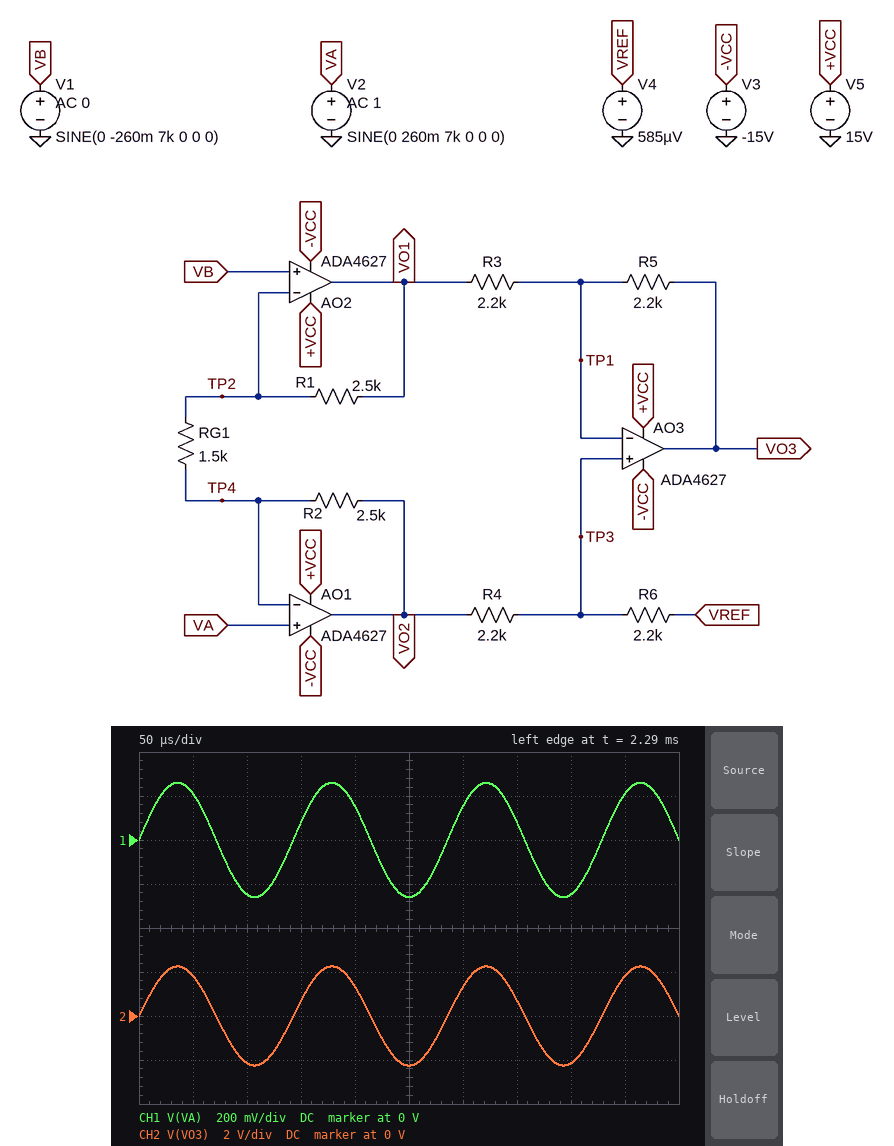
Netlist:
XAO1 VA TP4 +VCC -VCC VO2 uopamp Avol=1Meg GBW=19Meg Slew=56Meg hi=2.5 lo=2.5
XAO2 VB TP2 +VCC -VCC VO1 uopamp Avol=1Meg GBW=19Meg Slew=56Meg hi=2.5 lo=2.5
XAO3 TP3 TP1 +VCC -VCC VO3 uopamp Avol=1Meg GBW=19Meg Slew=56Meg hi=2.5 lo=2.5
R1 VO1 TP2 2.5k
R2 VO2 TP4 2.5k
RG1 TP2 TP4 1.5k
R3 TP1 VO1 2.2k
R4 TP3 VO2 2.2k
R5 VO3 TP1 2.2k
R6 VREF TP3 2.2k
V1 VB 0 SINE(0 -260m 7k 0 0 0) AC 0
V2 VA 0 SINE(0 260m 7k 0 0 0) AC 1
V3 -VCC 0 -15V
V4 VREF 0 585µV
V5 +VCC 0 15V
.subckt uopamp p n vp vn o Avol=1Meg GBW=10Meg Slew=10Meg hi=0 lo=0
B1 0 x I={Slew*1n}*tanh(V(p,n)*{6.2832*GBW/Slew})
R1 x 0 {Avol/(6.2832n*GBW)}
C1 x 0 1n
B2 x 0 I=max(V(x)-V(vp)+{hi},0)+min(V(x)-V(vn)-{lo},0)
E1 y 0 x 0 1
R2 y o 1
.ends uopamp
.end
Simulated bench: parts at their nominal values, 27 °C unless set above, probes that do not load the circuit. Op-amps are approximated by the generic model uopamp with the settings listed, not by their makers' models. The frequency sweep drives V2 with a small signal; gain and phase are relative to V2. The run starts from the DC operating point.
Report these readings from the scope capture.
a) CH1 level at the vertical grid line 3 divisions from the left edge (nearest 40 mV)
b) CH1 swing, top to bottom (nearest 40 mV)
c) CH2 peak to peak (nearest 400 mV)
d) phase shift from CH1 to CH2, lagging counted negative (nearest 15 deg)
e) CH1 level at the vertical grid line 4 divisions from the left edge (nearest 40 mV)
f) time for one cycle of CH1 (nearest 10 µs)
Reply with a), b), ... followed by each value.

a) 80 mV
b) 520 mV
c) 4.4 V
d) 0 deg
e) 160 mV
f) 140 µs
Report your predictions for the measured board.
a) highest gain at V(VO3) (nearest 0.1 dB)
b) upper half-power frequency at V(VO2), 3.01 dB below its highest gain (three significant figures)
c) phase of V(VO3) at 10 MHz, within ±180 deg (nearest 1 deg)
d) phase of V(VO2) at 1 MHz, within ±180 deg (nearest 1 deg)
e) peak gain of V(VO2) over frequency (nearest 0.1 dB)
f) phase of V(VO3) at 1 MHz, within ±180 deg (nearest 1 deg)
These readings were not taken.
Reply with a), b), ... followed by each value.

a) 12.7 dB
b) 4.79 MHz
c) -113 deg
d) -11 deg
e) 8.5 dB
f) -19 deg
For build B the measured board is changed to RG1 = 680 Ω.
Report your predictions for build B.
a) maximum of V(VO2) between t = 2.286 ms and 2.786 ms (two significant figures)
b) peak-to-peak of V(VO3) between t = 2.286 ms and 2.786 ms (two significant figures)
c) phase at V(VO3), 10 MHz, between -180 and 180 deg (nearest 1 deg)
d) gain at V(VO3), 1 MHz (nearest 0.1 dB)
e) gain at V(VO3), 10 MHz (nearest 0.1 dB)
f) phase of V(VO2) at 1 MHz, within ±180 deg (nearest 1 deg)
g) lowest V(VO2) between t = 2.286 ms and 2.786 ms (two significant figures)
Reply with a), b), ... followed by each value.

a) 2.2 V
b) 8.7 V
c) -124 deg
d) 17.6 dB
e) 2.1 dB
f) -21 deg
g) -2.2 V
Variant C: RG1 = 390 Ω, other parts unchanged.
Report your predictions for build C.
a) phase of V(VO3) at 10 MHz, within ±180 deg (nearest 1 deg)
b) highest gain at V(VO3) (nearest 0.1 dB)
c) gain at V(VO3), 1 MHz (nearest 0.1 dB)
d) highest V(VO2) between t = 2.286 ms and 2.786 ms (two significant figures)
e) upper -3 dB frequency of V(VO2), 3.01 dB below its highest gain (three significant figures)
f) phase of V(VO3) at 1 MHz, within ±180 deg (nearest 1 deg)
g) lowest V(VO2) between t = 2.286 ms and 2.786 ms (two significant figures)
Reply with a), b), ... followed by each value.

a) -129 deg
b) 22.8 dB
c) 20.9 dB
d) 3.6 V
e) 1.39 MHz
f) -42 deg
g) -3.6 V
